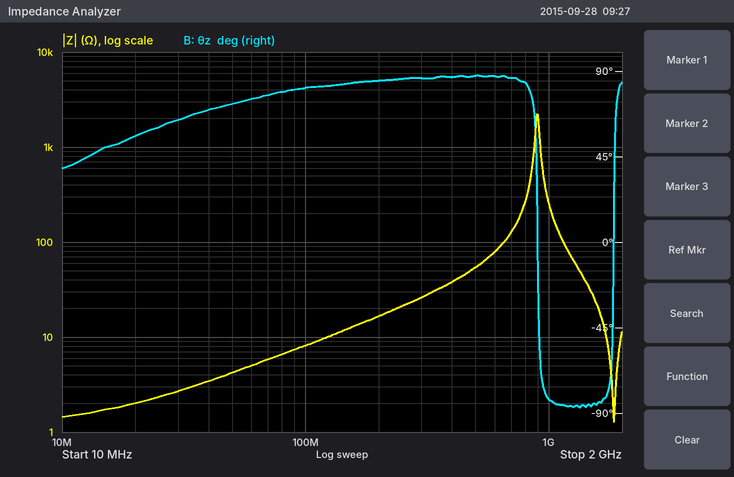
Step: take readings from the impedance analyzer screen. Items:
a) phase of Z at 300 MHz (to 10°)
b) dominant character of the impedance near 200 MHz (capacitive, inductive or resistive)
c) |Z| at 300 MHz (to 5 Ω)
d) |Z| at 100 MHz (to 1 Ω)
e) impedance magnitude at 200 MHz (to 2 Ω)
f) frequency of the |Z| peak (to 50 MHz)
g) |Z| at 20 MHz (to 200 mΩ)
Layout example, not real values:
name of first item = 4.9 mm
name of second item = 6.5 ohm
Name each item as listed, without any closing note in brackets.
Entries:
phase of Z at 300 MHz = 90°
dominant character of the impedance near 200 MHz = inductive
|Z| at 300 MHz = 25 Ω
|Z| at 100 MHz = 8 Ω
impedance magnitude at 200 MHz = 16 Ω
frequency of the |Z| peak = 900 MHz
|Z| at 20 MHz = 2.0 Ω
